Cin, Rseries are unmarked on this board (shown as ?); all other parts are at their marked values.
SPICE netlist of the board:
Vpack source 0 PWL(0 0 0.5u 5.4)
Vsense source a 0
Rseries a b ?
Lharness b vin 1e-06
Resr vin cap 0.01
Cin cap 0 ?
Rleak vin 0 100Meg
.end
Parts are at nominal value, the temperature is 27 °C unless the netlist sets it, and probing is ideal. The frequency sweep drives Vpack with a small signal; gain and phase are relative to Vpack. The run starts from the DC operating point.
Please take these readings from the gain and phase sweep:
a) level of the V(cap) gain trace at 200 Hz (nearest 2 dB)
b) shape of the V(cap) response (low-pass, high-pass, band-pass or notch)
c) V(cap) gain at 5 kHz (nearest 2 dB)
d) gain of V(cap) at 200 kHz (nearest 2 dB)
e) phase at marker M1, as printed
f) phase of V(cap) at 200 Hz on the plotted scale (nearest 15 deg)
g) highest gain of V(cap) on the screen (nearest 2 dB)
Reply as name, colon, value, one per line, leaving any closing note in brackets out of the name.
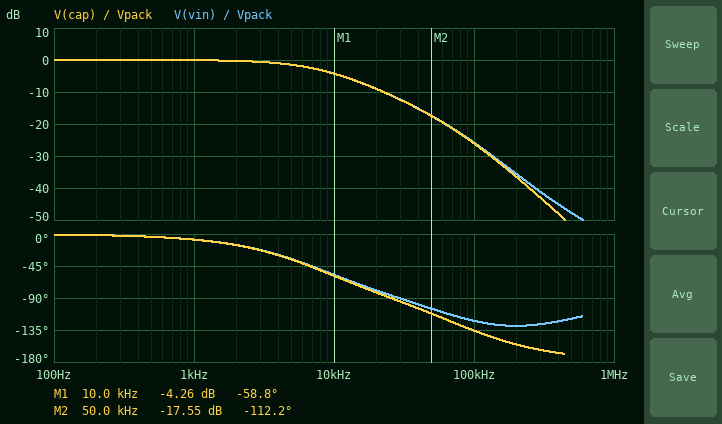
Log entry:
level of the V(cap) gain trace at 200 Hz: 0 dB
shape of the V(cap) response: low-pass
V(cap) gain at 5 kHz: -2 dB
gain of V(cap) at 200 kHz: -36 dB
phase at marker M1, as printed: -58.8 deg
phase of V(cap) at 200 Hz on the plotted scale: 0 deg
highest gain of V(cap) on the screen: 0 dB
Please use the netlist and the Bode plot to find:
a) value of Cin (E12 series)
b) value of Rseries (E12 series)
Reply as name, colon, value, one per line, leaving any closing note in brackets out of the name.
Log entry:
value of Cin: 39 µF
value of Rseries: 0.56 Ω
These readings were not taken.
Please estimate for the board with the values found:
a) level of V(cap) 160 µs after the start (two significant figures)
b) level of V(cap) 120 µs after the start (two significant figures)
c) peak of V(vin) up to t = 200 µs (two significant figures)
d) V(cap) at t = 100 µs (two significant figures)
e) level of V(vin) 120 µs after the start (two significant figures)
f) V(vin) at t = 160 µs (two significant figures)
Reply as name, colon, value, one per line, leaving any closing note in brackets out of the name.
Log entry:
level of V(cap) 160 µs after the start: 5.4 V
level of V(cap) 120 µs after the start: 5.4 V
peak of V(vin) up to t = 200 µs: 5.4 V
V(cap) at t = 100 µs: 5.4 V
level of V(vin) 120 µs after the start: 5.4 V
V(vin) at t = 160 µs: 5.4 V
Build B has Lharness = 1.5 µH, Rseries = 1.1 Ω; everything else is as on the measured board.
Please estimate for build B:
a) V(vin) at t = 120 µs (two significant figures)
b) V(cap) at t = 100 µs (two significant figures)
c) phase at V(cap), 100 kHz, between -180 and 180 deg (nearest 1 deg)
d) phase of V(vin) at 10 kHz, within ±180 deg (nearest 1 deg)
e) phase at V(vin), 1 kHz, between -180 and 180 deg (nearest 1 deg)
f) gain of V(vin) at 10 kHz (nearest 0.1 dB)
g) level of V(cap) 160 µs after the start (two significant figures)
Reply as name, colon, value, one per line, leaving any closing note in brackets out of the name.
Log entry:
V(vin) at t = 120 µs: 5.1 V
V(cap) at t = 100 µs: 4.9 V
phase at V(cap), 100 kHz, between -180 and 180 deg: -129 deg
phase of V(vin) at 10 kHz, within ±180 deg: -73 deg
phase at V(vin), 1 kHz, between -180 and 180 deg: -15 deg
gain of V(vin) at 10 kHz: -9.0 dB
level of V(cap) 160 µs after the start: 5.3 V
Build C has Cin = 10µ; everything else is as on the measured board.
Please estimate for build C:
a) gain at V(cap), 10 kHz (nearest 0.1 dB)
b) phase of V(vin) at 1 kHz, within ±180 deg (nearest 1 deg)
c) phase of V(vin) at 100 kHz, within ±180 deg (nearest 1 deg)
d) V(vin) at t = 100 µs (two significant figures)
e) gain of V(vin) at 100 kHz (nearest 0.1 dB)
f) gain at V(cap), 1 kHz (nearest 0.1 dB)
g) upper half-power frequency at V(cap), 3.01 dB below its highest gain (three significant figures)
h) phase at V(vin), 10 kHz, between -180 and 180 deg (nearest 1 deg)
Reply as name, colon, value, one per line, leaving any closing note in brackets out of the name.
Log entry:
gain at V(cap), 10 kHz: -0.2 dB
phase of V(vin) at 1 kHz, within ±180 deg: -2 deg
phase of V(vin) at 100 kHz, within ±180 deg: -126 deg
V(vin) at t = 100 µs: 5.4 V
gain of V(vin) at 100 kHz: -13.3 dB
gain at V(cap), 1 kHz: 0 dB
upper half-power frequency at V(cap), 3.01 dB below its highest gain: 37.5 kHz
phase at V(vin), 10 kHz, between -180 and 180 deg: -20 deg
